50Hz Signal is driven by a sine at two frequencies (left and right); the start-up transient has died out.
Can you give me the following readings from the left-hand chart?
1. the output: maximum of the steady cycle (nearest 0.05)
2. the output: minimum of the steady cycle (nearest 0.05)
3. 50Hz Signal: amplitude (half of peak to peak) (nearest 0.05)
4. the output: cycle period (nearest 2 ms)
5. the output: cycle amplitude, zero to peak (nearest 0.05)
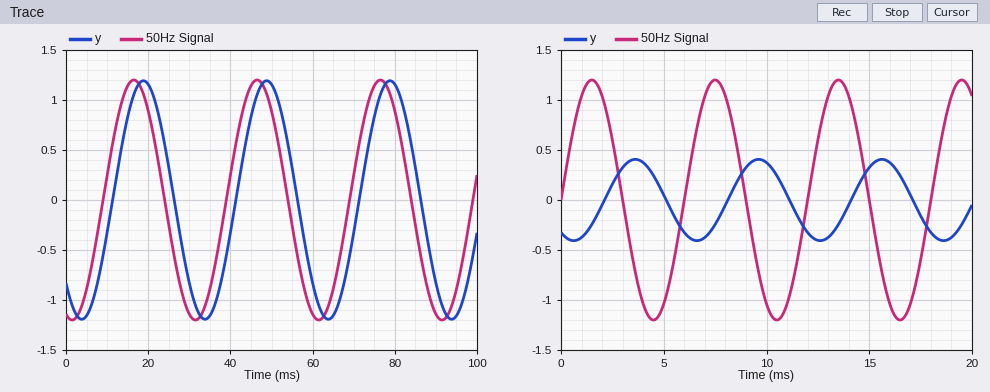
1.20
-1.20
1.20
30 ms
1.20
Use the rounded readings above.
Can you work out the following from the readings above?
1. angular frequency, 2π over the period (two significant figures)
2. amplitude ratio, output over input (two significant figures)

0.21 rad/ms
1.0
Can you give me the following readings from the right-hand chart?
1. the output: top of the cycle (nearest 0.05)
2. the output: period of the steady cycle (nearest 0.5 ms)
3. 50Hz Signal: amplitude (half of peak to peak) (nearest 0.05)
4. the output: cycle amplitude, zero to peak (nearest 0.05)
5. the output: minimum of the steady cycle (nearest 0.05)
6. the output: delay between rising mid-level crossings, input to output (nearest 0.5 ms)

0.40
6.0 ms
1.20
0.40
-0.40
2.0 ms
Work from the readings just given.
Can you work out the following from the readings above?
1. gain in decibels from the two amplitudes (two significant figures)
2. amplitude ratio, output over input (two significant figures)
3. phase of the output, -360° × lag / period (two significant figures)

-9.5 dB
0.33
-120°
